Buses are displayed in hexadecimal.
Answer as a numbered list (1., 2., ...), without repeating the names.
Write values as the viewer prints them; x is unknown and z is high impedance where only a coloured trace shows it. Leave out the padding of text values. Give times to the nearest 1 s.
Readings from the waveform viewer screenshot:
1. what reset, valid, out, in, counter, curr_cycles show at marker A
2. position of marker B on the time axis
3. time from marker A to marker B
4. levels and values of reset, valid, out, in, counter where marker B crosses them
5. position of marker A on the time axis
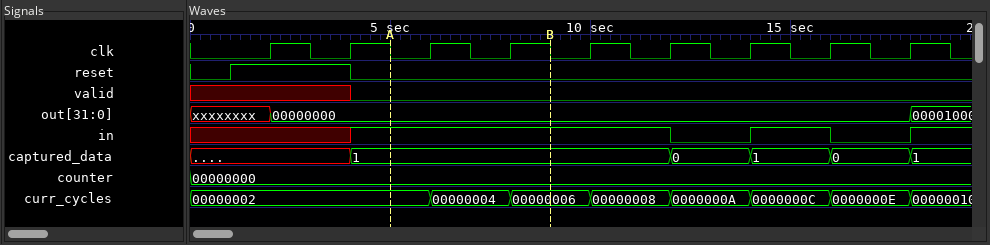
1. reset=0, valid=0, out=00000000, in=1, counter=00000000, curr_cycles=00000002
2. 9 s
3. 4 s
4. reset=0, valid=0, out=00000000, in=1, counter=00000000
5. 5 s
